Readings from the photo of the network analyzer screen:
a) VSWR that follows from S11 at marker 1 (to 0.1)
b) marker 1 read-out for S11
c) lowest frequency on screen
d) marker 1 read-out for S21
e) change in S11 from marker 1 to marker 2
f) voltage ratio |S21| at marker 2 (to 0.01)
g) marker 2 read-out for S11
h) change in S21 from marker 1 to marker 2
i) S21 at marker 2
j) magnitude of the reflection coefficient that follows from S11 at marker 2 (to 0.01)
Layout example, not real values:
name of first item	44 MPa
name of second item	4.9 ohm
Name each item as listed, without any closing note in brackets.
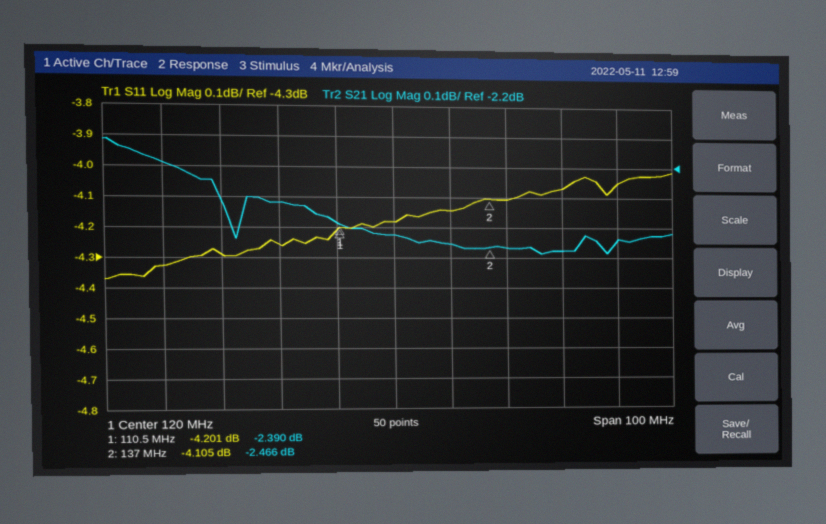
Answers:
VSWR that follows from S11 at marker 1	4.2
marker 1 read-out for S11	-4.201 dB
lowest frequency on screen	70 MHz
marker 1 read-out for S21	-2.390 dB
change in S11 from marker 1 to marker 2	0.096 dB
voltage ratio |S21| at marker 2	0.75
marker 2 read-out for S11	-4.105 dB
change in S21 from marker 1 to marker 2	-0.076 dB
S21 at marker 2	-2.466 dB
magnitude of the reflection coefficient that follows from S11 at marker 2	0.62
